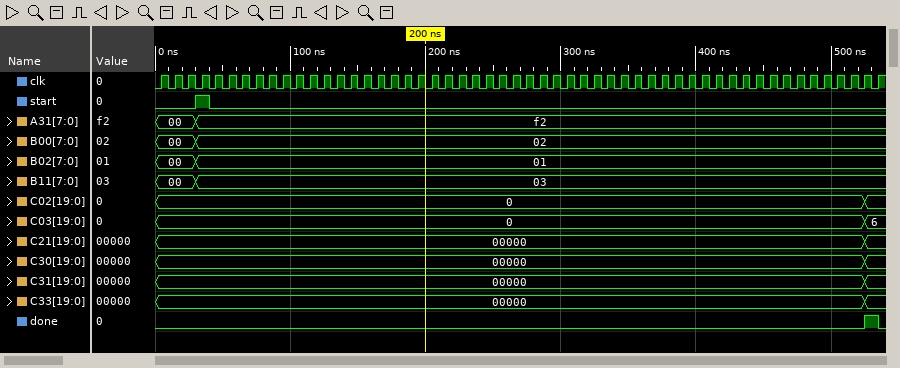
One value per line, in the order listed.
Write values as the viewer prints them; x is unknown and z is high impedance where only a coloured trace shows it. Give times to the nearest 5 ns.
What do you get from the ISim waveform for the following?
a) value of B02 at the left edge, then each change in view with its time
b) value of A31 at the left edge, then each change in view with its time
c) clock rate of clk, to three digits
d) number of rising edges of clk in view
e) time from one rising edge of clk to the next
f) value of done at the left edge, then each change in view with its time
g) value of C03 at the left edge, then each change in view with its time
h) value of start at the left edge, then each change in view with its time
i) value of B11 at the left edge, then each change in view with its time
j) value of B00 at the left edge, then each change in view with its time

00, 01 at 30 ns
00, f2 at 30 ns
100 MHz
54
10 ns
0, 1 at 525 ns, 0 at 535 ns
0, 6 at 525 ns
0, 1 at 30 ns, 0 at 40 ns
00, 03 at 30 ns
00, 02 at 30 ns
